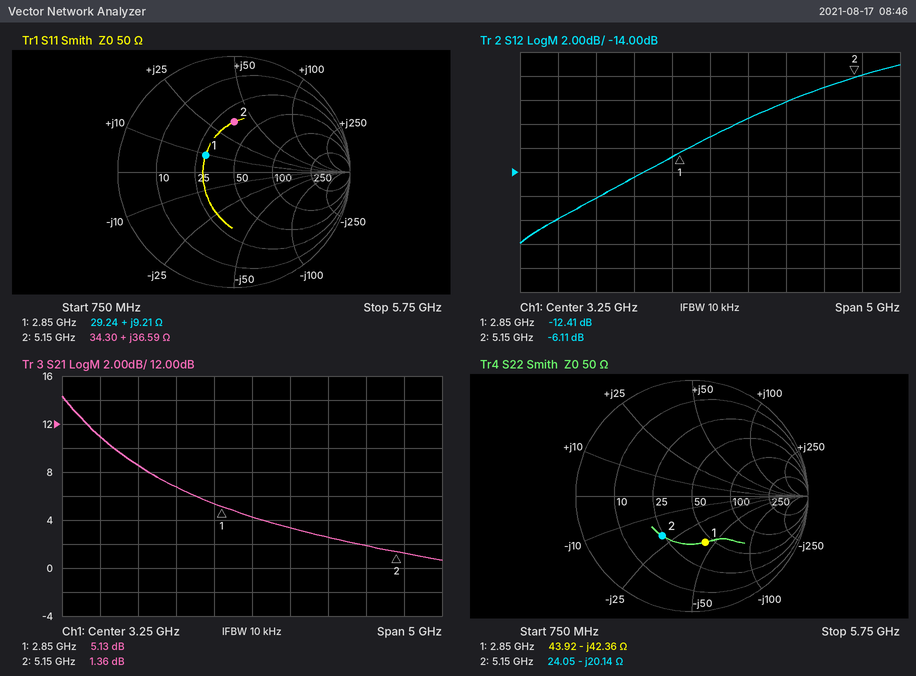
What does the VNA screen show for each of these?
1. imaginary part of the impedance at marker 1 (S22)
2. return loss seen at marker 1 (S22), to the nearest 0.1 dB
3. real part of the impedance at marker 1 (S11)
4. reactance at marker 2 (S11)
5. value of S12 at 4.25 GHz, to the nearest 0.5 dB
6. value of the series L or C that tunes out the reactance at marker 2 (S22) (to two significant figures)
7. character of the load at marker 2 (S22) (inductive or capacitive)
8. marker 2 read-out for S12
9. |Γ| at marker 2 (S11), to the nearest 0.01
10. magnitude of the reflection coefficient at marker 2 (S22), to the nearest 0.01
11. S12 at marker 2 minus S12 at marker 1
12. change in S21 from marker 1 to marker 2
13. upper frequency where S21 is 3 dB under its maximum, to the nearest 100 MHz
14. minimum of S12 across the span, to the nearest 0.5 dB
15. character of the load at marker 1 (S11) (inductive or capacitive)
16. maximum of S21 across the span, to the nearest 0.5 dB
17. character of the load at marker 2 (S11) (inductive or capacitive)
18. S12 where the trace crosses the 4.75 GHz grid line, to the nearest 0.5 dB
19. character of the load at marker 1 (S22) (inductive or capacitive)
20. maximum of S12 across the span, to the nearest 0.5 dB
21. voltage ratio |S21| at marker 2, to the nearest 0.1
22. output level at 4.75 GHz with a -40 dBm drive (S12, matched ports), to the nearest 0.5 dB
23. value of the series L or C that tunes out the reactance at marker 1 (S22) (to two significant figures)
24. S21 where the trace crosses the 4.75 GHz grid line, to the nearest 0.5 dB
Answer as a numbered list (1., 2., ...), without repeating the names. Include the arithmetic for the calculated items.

1. -42.36 Ω
2. 7.6 dB
3. 29.24 Ω
4. +36.59 Ω
5. -8.0 dB
6. L = 20.14 Ω/(2π × 5.15 GHz) ≈ 622 pH, so 620 pH to two significant figures
7. capacitive
8. -6.11 dB
9. 0.43
10. 0.43
11. -6.11 − (-12.41) = 6.30 dB
12. 1.36 − (5.13) = -3.77 dB
13. 1.2 GHz
14. -20.0 dB
15. inductive
16. 14.5 dB
17. inductive
18. -7.0 dB
19. capacitive
20. -5.0 dB
21. 10^(1.36/20) ≈ 1.2
22. -40 dBm + (-7.0 dB) = -47.0 dBm
23. L = 42.36 Ω/(2π × 2.85 GHz) ≈ 2.4 nH
24. 2.0 dB
